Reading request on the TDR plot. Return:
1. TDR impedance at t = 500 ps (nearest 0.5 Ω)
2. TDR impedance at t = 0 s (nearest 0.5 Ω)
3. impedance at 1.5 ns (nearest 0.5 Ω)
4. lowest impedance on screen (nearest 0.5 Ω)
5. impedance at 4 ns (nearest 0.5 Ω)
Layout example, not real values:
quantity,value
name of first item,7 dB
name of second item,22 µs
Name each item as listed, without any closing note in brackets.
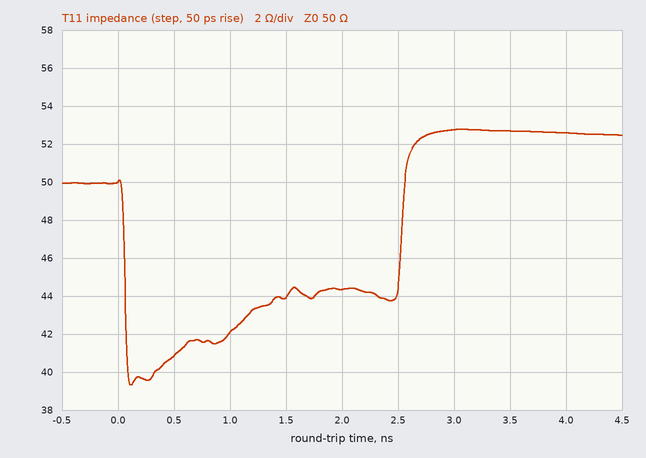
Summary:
quantity,value
TDR impedance at t = 500 ps,41.0 Ω
TDR impedance at t = 0 s,50.0 Ω
impedance at 1.5 ns,44.0 Ω
lowest impedance on screen,39.5 Ω
impedance at 4 ns,52.5 Ω
